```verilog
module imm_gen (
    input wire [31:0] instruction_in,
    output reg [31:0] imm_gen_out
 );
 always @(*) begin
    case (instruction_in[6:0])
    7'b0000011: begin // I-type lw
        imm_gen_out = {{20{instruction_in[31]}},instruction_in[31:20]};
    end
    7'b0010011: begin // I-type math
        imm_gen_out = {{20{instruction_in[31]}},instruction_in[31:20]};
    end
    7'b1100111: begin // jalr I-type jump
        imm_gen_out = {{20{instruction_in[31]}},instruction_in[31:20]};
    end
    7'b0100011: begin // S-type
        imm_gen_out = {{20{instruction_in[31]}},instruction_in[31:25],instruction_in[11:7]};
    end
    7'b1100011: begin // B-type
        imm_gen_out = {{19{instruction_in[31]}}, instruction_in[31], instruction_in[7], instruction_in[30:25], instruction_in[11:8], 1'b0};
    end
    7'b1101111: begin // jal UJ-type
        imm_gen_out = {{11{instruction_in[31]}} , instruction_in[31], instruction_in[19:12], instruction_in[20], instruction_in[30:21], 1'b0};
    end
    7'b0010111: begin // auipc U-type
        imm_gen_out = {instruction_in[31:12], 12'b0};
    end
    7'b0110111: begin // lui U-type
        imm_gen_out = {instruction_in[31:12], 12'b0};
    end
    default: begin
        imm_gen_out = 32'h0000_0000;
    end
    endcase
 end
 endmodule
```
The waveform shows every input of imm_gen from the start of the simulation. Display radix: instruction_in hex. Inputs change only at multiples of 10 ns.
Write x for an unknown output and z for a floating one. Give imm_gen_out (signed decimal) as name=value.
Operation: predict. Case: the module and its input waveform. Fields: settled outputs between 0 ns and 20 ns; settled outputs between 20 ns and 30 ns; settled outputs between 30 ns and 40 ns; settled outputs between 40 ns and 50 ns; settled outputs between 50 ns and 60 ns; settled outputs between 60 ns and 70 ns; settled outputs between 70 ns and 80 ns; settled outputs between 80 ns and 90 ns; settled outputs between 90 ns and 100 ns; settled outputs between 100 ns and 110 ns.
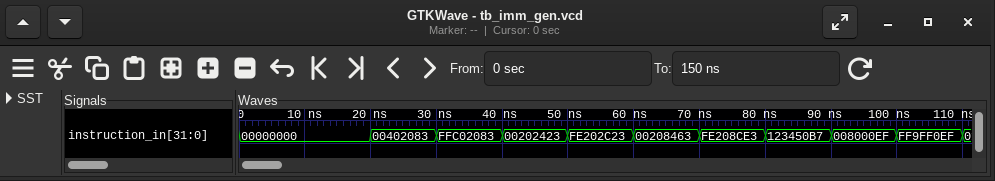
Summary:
imm_gen_out=0
imm_gen_out=4
imm_gen_out=-4
imm_gen_out=8
imm_gen_out=-8
imm_gen_out=8
imm_gen_out=-8
imm_gen_out=305418240
imm_gen_out=8
imm_gen_out=-8
